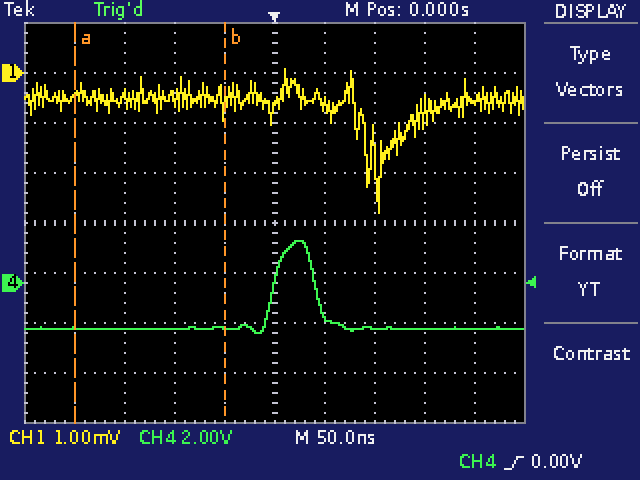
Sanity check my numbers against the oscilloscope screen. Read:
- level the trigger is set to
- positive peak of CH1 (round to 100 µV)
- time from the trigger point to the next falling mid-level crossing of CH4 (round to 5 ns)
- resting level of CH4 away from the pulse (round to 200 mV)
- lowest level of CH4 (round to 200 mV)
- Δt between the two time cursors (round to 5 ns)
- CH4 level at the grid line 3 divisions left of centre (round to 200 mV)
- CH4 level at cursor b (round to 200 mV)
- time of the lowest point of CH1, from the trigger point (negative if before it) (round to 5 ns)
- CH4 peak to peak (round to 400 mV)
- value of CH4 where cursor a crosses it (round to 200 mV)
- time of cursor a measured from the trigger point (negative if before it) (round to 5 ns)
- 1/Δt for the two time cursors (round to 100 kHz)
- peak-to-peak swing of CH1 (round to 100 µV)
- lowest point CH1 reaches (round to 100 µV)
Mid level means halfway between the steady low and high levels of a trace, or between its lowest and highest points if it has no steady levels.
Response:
0.00 V
100 µV
40 ns
-1.8 V
-2.0 V
150 ns
-1.8 V
-1.8 V
+105 ns
3.6 V
-1.8 V
-200 ns
6.7 MHz
2.9 mV
-2.8 mV
